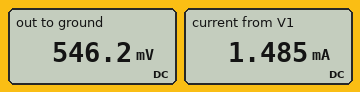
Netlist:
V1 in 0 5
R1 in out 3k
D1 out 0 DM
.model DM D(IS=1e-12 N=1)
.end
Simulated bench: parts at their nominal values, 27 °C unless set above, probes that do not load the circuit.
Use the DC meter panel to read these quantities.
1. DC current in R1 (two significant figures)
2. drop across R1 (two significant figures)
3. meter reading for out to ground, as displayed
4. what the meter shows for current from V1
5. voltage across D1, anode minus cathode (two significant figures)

1.5 mA
4.5 V
546.2 mV
1.485 mA
550 mV
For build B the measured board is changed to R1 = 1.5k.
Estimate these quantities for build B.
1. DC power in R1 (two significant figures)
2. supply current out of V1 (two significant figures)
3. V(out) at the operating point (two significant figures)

13 mW
3.0 mA
560 mV
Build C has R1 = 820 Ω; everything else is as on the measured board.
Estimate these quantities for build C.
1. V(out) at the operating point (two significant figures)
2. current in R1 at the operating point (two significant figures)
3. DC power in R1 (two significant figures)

580 mV
5.4 mA
24 mW
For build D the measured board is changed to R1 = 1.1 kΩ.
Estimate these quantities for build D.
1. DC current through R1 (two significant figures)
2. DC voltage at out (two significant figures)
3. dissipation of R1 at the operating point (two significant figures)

4.0 mA
570 mV
18 mW
